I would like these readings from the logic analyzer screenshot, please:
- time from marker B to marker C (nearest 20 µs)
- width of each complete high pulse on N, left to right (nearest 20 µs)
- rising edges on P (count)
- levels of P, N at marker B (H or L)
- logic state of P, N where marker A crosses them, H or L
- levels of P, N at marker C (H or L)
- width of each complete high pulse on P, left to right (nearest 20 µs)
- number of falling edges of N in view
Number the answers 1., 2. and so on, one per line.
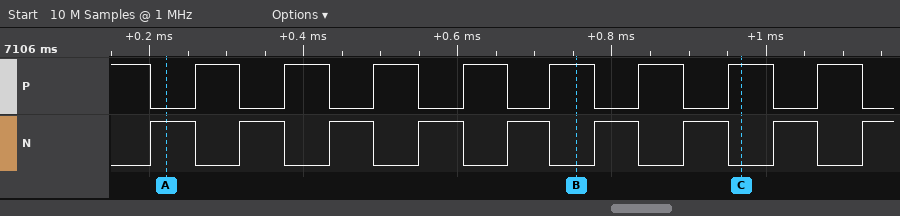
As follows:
1. 220 µs
2. 60 µs, 60 µs, 60 µs, 60 µs, 60 µs, 60 µs, 60 µs, 60 µs
3. 8
4. P=H, N=L
5. P=L, N=H
6. P=H, N=L
7. 60 µs, 60 µs, 60 µs, 60 µs, 60 µs, 60 µs, 60 µs, 60 µs
8. 8
